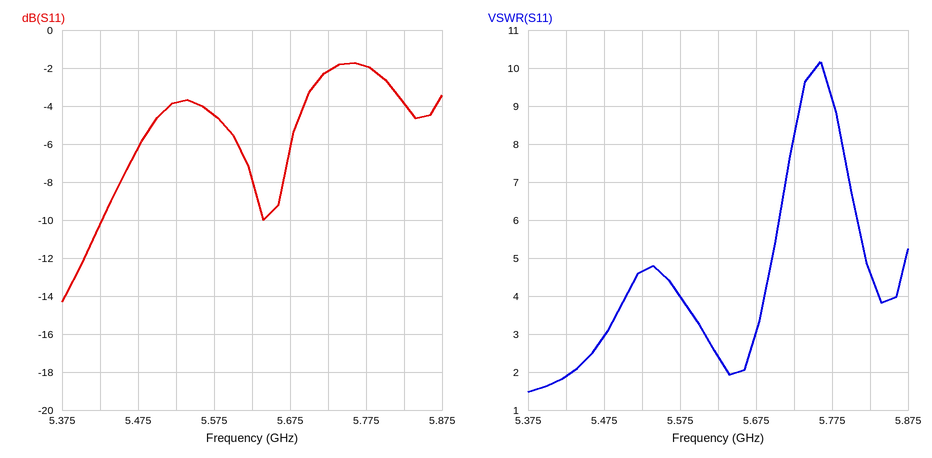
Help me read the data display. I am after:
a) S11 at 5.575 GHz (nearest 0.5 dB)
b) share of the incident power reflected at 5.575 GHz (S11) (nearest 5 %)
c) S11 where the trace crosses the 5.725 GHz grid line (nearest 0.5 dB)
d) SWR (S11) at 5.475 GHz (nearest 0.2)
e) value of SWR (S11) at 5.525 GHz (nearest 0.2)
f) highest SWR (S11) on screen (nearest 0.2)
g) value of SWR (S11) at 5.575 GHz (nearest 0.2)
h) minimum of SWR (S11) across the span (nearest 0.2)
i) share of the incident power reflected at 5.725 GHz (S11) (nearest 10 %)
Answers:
-4.5 dB
35 %
-2.0 dB
3.0
4.6
10.2
4.0
1.4
60 %
